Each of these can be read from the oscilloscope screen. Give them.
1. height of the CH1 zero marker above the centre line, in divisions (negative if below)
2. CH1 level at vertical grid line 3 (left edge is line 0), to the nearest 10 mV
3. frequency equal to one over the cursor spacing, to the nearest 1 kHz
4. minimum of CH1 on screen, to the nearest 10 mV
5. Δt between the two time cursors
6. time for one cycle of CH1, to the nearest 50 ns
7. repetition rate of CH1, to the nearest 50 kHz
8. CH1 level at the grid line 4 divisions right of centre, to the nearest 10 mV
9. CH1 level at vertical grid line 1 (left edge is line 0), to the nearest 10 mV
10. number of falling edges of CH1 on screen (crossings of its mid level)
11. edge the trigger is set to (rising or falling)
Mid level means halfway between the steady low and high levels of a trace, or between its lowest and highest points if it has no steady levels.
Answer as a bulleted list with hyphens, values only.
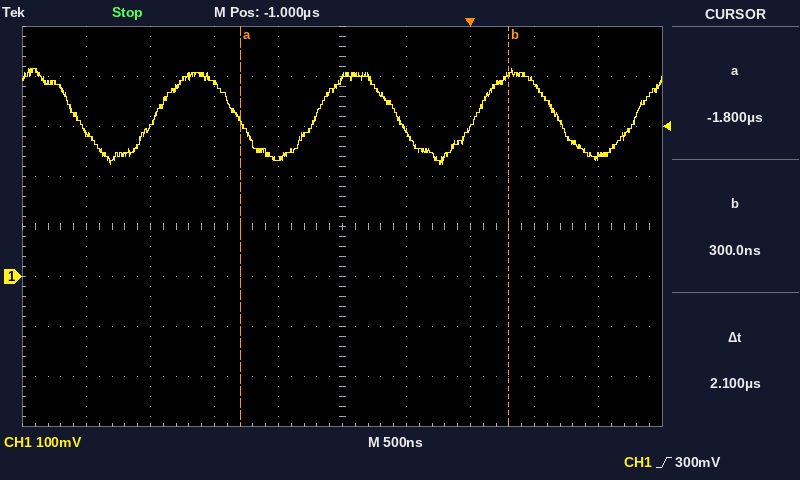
- -1.0 div
- 390 mV
- 476 kHz
- 220 mV
- 2.1 µs
- 1.25 µs
- 800 kHz
- 240 mV
- 290 mV
- 4
- rising
